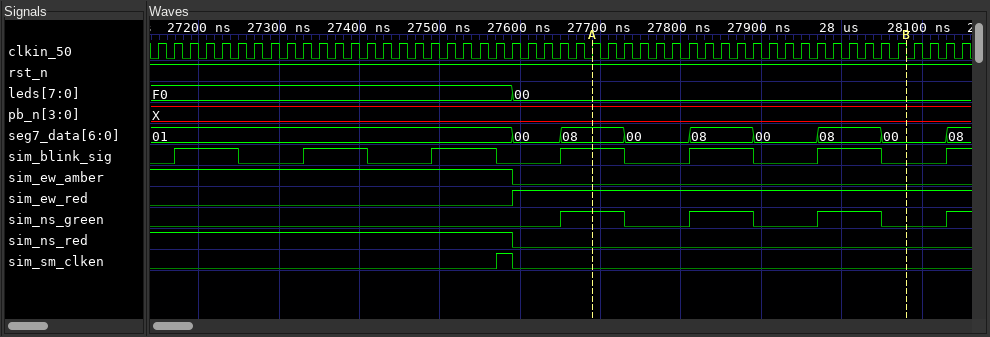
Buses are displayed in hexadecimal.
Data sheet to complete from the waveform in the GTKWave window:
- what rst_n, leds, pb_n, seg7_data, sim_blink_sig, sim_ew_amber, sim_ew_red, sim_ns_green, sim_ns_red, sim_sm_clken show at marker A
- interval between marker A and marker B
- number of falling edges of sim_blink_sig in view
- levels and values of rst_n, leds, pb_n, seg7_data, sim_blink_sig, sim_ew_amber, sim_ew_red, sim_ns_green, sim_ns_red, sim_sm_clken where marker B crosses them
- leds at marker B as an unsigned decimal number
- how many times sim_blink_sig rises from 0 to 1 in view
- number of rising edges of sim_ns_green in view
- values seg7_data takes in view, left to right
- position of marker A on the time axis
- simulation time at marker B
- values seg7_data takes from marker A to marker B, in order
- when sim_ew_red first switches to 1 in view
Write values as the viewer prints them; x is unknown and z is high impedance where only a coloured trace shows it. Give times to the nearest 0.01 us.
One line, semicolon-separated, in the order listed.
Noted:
rst_n=1, leds=00, pb_n=X, seg7_data=08, sim_blink_sig=1, sim_ew_amber=0, sim_ew_red=1, sim_ns_green=1, sim_ns_red=0, sim_sm_clken=0; 0.39 us; 6; rst_n=1, leds=00, pb_n=X, seg7_data=00, sim_blink_sig=0, sim_ew_amber=0, sim_ew_red=1, sim_ns_green=0, sim_ns_red=0, sim_sm_clken=0; 0; 7; 4; 01, 00, 08, 00, 08, 00, 08, 00, 08; 27.69 us; 28.08 us; 08, 00, 08, 00, 08, 00; 27.59 us
